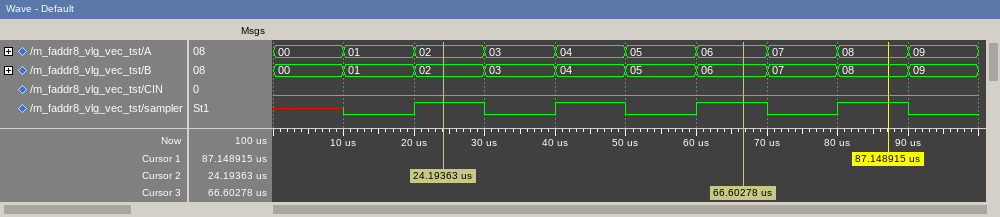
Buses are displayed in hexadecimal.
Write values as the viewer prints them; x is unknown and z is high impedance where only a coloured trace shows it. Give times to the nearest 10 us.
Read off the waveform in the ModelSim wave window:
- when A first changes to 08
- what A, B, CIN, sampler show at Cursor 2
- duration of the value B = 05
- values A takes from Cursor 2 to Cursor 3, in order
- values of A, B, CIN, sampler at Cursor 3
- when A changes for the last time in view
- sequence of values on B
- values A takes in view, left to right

80 us
A=02, B=02, CIN=0, sampler=1
10 us
02, 03, 04, 05, 06
A=06, B=06, CIN=0, sampler=1
90 us
00, 01, 02, 03, 04, 05, 06, 07, 08, 09
00, 01, 02, 03, 04, 05, 06, 07, 08, 09
